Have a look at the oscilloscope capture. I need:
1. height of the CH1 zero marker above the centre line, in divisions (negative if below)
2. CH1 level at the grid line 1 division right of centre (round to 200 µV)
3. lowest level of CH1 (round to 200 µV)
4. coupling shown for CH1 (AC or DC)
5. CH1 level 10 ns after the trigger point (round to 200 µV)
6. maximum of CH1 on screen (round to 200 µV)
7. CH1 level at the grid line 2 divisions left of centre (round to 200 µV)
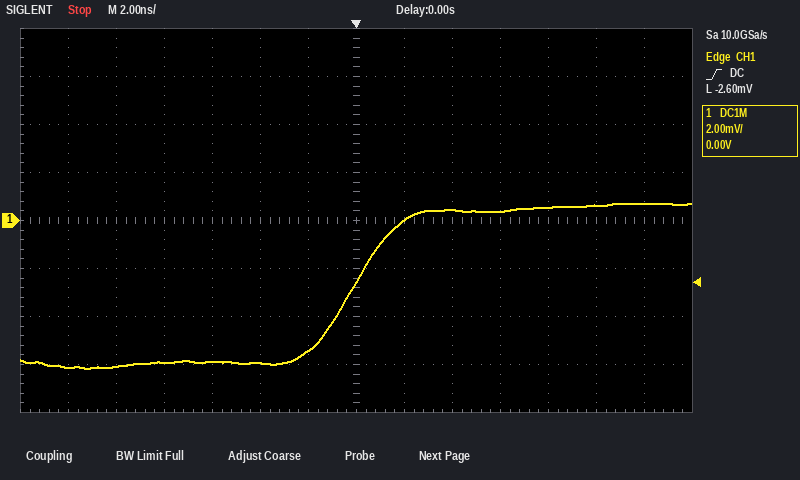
0.0 div
0.0 mV
-6.2 mV
DC
600 µV
800 µV
-6.0 mV
